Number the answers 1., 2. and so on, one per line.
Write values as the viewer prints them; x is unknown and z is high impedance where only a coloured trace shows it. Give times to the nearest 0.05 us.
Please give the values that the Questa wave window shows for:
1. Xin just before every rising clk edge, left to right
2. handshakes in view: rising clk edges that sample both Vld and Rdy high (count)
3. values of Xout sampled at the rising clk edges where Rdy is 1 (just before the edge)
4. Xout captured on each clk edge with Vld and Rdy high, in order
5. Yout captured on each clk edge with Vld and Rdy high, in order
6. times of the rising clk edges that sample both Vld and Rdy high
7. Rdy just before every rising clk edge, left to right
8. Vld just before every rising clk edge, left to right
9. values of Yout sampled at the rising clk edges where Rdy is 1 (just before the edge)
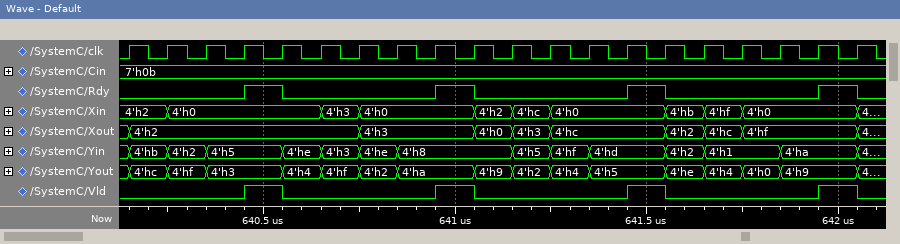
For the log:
1. 4'h2, 4'h2, 4'h0, 4'h0, 4'h0, 4'h0, 4'h3, 4'h0, 4'h0, 4'h0, 4'h2, 4'hc, 4'h0, 4'h0, 4'h0, 4'hb, 4'hf, 4'h0, 4'h0, 4'h0
2. 4
3. 4'h2, 4'h3, 4'hc, 4'hf
4. 4'h2, 4'h3, 4'hc, 4'hf
5. 4'h3, 4'ha, 4'h5, 4'h9
6. 640.55 us, 641.05 us, 641.55 us, 642.05 us
7. 0 0 0 0 1 0 0 0 0 1 0 0 0 0 1 0 0 0 0 1
8. 0 0 0 0 1 0 0 0 0 1 0 0 0 0 1 0 0 0 0 1
9. 4'h3, 4'ha, 4'h5, 4'h9
